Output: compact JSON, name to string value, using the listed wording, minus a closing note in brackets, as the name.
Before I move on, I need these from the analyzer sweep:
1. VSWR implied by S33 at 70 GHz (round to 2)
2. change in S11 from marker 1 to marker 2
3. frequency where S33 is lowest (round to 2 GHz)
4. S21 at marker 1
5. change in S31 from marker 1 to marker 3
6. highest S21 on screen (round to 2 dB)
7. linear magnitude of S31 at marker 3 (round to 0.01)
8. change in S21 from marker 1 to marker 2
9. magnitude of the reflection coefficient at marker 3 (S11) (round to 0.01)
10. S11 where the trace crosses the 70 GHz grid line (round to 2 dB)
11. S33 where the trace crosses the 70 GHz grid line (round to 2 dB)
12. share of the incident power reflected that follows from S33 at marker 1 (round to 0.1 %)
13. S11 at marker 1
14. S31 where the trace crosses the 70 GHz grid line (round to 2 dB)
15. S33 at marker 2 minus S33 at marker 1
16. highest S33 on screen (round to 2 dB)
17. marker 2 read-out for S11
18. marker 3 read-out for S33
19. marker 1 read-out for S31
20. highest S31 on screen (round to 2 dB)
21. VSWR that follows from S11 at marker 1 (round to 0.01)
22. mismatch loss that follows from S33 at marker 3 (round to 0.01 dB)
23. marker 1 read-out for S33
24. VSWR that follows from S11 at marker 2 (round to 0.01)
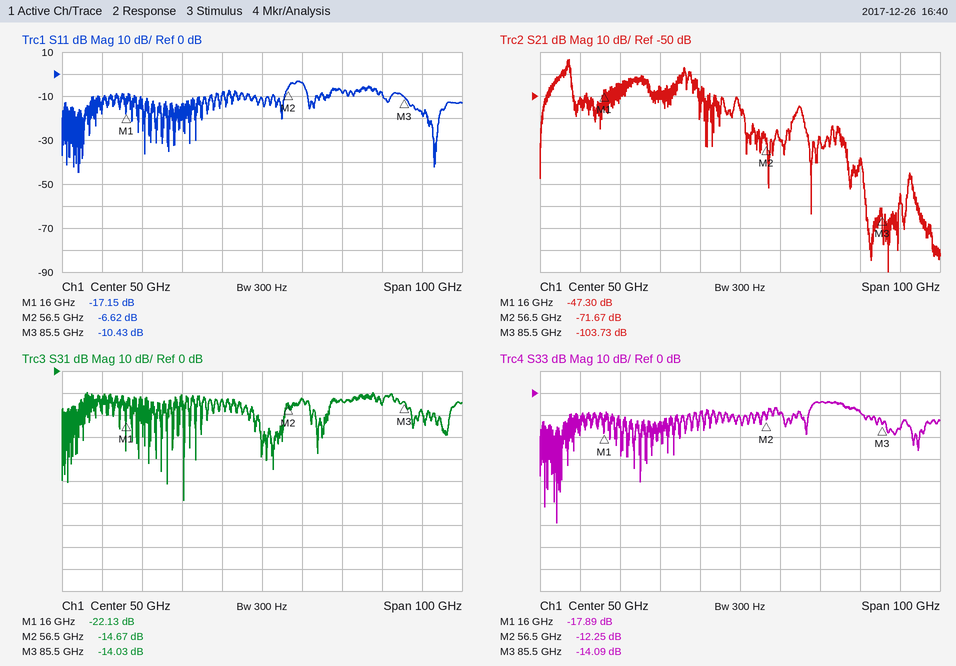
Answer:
{"VSWR implied by S33 at 70 GHz": "4", "change in S11 from marker 1 to marker 2": "10.53 dB", "frequency where S33 is lowest": "4 GHz", "S21 at marker 1": "-47.30 dB", "change in S31 from marker 1 to marker 3": "8.10 dB", "highest S21 on screen": "-34 dB", "linear magnitude of S31 at marker 3": "0.20", "change in S21 from marker 1 to marker 2": "-24.37 dB", "magnitude of the reflection coefficient at marker 3 (S11)": "0.30", "S11 where the trace crosses the 70 GHz grid line": "-8 dB", "S33 where the trace crosses the 70 GHz grid line": "-4 dB", "share of the incident power reflected that follows from S33 at marker 1": "1.6 %", "S11 at marker 1": "-17.15 dB", "S31 where the trace crosses the 70 GHz grid line": "-14 dB", "S33 at marker 2 minus S33 at marker 1": "5.64 dB", "highest S33 on screen": "-4 dB", "marker 2 read-out for S11": "-6.62 dB", "marker 3 read-out for S33": "-14.09 dB", "marker 1 read-out for S31": "-22.13 dB", "highest S31 on screen": "-10 dB", "VSWR that follows from S11 at marker 1": "1.32", "mismatch loss that follows from S33 at marker 3": "0.17 dB", "marker 1 read-out for S33": "-17.89 dB", "VSWR that follows from S11 at marker 2": "2.75"}
